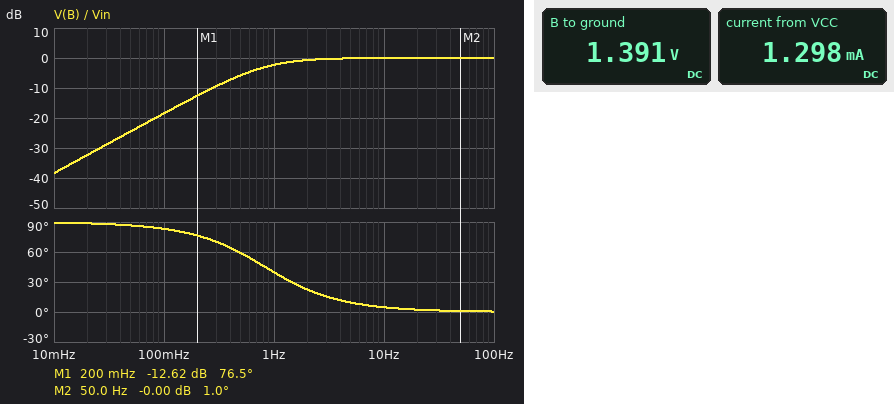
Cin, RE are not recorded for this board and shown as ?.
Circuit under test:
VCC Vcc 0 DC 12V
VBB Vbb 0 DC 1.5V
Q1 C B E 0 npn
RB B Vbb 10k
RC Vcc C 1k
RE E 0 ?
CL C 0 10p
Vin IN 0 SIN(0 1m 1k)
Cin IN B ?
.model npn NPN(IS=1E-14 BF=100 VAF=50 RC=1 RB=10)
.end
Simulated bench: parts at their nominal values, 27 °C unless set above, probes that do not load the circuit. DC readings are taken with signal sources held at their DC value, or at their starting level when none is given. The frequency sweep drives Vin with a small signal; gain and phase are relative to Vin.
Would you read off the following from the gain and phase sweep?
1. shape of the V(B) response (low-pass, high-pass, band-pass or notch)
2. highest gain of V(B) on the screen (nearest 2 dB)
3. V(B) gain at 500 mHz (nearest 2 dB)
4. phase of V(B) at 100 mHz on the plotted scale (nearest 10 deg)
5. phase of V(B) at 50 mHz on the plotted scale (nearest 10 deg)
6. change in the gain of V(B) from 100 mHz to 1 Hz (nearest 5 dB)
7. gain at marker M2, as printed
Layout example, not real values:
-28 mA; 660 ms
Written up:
high-pass; 0 dB; -6 dB; 80 deg; 90 deg; 15 dB; -0.00 dB
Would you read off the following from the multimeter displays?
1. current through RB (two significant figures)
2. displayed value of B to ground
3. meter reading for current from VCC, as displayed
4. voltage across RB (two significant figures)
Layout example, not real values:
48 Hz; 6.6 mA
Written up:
11 µA; 1.391 V; 1.298 mA; 110 mV
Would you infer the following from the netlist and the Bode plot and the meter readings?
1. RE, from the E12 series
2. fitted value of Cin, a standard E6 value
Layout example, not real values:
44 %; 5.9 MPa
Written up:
560 Ω; 22 µF
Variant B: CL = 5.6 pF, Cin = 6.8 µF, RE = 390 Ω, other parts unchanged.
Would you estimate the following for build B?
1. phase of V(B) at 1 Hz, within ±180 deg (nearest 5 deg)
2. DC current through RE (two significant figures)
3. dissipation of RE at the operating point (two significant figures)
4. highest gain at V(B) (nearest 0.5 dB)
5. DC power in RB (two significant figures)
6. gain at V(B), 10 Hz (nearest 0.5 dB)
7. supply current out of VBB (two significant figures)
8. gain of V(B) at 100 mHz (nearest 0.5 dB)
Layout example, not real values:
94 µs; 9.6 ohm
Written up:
70 deg; 1.8 mA; 1.2 mW; 0 dB; 2.2 µW; -0.5 dB; 15 µA; -29.0 dB
